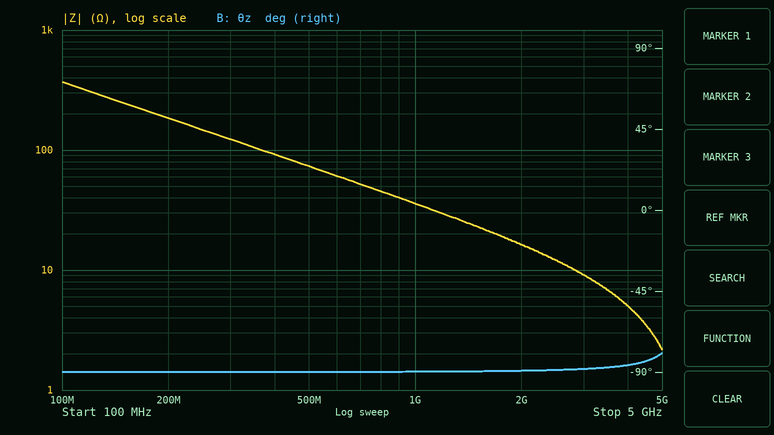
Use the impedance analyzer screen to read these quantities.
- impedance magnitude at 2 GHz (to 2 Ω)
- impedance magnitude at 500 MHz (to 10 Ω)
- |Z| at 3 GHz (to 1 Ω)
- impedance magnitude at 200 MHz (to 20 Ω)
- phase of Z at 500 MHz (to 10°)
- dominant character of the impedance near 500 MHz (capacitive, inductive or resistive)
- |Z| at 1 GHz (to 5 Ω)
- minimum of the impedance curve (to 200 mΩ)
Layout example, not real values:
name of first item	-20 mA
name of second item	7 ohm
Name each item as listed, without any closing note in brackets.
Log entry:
impedance magnitude at 2 GHz	16 Ω
impedance magnitude at 500 MHz	70 Ω
|Z| at 3 GHz	9 Ω
impedance magnitude at 200 MHz	180 Ω
phase of Z at 500 MHz	-90°
dominant character of the impedance near 500 MHz	capacitive
|Z| at 1 GHz	35 Ω
minimum of the impedance curve	2.2 Ω
